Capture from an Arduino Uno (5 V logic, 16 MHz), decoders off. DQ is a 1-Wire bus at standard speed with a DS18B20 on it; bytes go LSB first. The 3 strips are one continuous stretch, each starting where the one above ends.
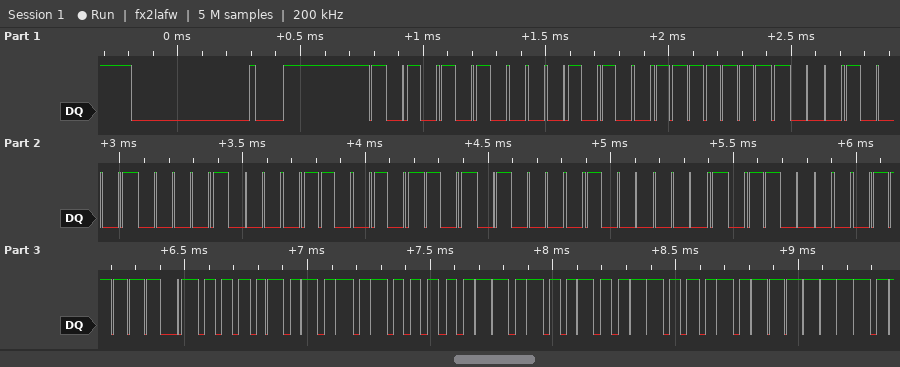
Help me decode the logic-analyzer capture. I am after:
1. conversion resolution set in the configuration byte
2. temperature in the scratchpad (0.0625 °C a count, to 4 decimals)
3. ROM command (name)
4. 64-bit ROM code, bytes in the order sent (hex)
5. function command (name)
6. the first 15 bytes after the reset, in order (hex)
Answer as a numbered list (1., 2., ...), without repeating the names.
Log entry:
1. 12 bits
2. 85.0000 °C
3. Match ROM
4. 28 FF 88 10 A6 15 02 0D
5. Read Scratchpad
6. 55 28 FF 88 10 A6 15 02 0D BE 50 05 4B 46 7F
